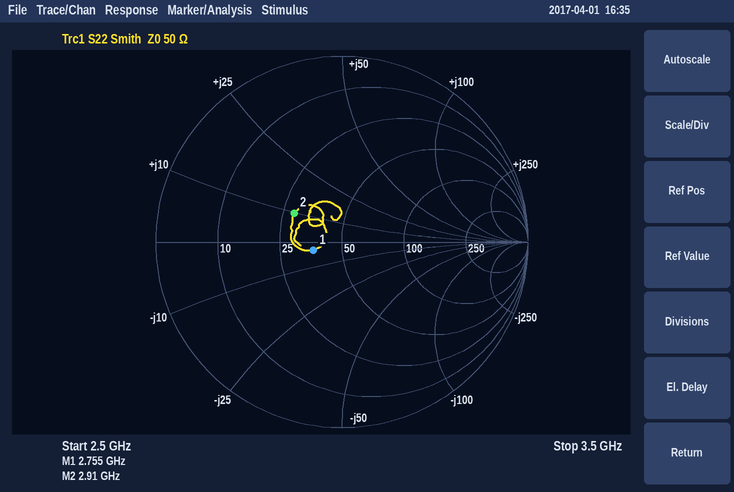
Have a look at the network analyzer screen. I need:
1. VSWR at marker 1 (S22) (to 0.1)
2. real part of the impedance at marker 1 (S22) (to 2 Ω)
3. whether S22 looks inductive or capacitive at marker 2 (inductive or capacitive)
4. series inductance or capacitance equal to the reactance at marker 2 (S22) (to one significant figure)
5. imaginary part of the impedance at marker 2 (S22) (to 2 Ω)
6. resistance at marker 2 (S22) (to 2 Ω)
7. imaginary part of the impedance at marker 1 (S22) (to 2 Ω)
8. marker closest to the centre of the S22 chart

1.4
36 Ω
inductive
500 pH
+10 Ω
28 Ω
-4 Ω
marker 1
